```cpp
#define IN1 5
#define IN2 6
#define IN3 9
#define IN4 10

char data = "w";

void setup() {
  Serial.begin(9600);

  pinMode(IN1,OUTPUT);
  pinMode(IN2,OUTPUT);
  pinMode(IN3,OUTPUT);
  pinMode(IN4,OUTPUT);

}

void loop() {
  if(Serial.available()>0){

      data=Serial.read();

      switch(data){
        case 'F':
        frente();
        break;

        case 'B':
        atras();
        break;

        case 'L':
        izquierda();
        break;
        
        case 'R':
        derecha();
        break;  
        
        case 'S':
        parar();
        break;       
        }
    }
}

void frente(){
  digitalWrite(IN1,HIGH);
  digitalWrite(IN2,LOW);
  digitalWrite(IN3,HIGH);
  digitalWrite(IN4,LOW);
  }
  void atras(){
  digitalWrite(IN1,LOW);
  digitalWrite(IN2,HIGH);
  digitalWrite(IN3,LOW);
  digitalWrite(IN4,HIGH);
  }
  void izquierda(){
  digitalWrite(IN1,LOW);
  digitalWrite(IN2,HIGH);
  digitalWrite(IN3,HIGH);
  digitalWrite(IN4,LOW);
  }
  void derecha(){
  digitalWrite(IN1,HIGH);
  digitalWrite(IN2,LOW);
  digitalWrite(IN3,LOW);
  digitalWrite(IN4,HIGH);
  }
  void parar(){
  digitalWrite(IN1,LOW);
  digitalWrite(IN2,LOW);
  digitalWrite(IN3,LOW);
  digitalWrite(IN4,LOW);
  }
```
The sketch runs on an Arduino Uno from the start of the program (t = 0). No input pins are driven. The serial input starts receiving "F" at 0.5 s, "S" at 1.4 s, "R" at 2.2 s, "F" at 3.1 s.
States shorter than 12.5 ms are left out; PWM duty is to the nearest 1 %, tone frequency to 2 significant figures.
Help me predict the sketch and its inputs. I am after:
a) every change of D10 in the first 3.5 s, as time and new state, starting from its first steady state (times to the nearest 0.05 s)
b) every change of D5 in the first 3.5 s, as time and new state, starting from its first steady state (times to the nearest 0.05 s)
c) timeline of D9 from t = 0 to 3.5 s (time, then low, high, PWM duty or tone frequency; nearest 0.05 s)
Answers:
0 s low; 2.2 s high; 3.1 s low
0 s low; 0.5 s high; 1.4 s low; 2.2 s high
0 s low; 0.5 s high; 1.4 s low; 3.1 s high
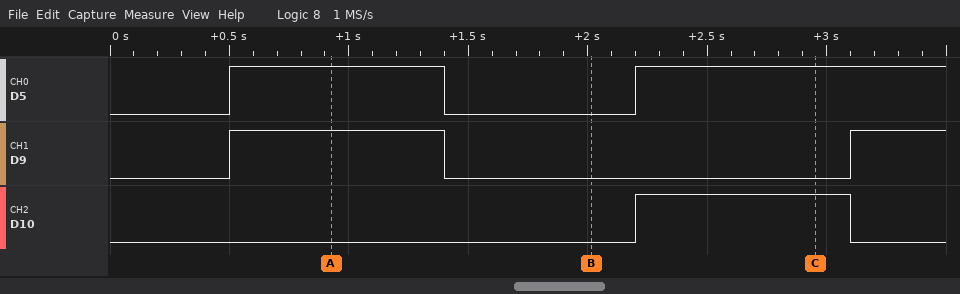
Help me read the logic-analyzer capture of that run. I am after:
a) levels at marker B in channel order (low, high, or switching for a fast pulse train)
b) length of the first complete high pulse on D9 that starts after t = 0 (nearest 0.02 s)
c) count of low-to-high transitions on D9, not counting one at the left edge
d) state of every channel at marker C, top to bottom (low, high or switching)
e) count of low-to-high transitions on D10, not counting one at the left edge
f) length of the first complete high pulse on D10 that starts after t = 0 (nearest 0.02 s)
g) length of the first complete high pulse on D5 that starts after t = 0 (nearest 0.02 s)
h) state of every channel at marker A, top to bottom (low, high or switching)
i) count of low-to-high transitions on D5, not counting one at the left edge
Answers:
D5 low, D9 low, D10 low
0.90 s
2
D5 high, D9 low, D10 high
1
0.90 s
0.90 s
D5 high, D9 high, D10 low
2
